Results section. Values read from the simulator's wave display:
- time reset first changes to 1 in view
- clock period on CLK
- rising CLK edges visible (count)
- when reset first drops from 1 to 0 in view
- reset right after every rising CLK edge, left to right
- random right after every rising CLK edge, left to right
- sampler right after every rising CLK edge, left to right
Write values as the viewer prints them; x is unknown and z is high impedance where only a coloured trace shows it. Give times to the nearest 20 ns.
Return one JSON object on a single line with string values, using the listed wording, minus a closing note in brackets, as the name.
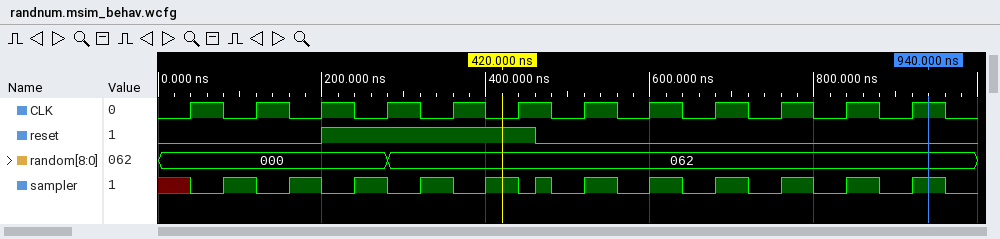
{"time reset first changes to 1 in view": "200 ns", "clock period on CLK": "80 ns", "rising CLK edges visible": "12", "when reset first drops from 1 to 0 in view": "460 ns", "reset right after every rising CLK edge, left to right": "0 0 1 1 1 1 0 0 0 0 0 0", "random right after every rising CLK edge, left to right": "000, 000, 000, 062, 062, 062, 062, 062, 062, 062, 062, 062", "sampler right after every rising CLK edge, left to right": "0 0 0 0 0 0 1 1 1 1 1 1"}
